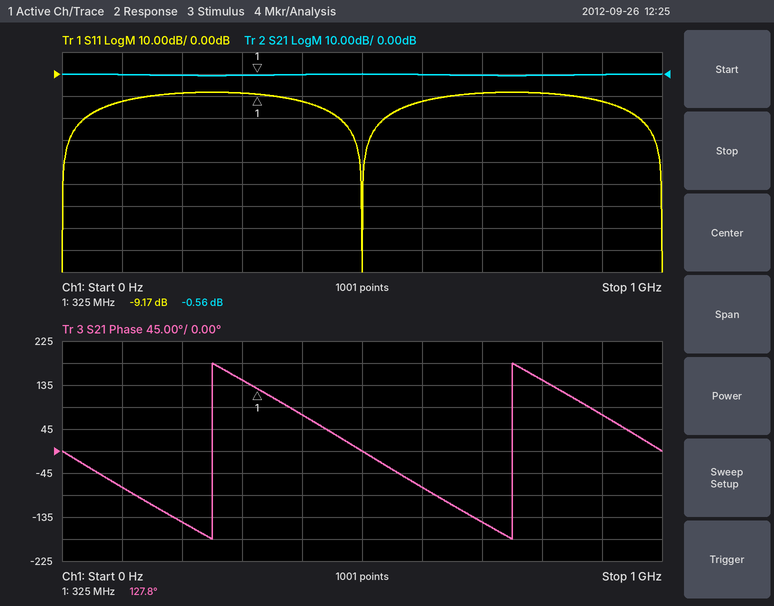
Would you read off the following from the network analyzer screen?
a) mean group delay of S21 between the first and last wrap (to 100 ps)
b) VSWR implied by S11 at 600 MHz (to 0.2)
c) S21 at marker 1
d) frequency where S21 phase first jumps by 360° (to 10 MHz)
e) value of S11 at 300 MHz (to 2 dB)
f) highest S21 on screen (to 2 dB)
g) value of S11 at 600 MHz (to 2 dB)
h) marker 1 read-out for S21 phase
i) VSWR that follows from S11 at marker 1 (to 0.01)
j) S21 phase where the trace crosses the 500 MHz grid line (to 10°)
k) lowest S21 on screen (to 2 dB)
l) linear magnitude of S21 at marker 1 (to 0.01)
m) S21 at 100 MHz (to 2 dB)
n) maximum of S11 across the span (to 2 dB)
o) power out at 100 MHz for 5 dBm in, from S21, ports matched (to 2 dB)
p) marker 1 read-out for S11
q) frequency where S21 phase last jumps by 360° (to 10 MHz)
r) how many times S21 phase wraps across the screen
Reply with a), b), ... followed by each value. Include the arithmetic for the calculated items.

a) 1 cycle / (750 MHz − 250 MHz) ≈ 2.0 ns
b) |Γ| = 10^(-12/20) = 0.2512; VSWR = (1 + 0.2512)/(1 − 0.2512) ≈ 1.67, so 1.6 to the nearest 0.2
c) -0.56 dB
d) 250 MHz
e) -8 dB
f) 0 dB
g) -12 dB
h) 127.8°
i) (1 + 0.3479)/(1 − 0.3479) ≈ 2.07
j) 0°
k) 0 dB
l) 10^(-0.56/20) ≈ 0.94
m) 0 dB
n) -8 dB
o) 5 dBm + (0 dB) = 4 dBm
p) -9.17 dB
q) 750 MHz
r) 2
